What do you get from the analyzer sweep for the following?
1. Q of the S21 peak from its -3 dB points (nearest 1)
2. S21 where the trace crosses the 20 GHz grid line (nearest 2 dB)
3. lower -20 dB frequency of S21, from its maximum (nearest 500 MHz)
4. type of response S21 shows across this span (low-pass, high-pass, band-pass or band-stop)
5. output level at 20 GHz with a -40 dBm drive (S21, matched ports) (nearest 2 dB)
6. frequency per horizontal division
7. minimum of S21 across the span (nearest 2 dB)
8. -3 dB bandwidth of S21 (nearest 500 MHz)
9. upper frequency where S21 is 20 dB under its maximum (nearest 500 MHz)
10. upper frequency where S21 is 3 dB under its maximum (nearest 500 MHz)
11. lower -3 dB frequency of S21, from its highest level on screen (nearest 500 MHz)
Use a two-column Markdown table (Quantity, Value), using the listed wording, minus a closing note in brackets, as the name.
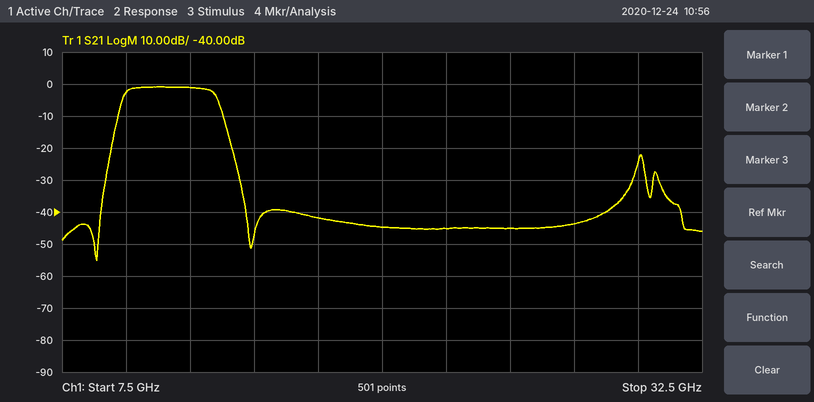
| Quantity | Value |
|---|---|
| Q of the S21 peak from its -3 dB points | 3 |
| S21 where the trace crosses the 20 GHz grid line | -44 dB |
| lower -20 dB frequency of S21, from its maximum | 9.5 GHz |
| type of response S21 shows across this span | band-pass |
| output level at 20 GHz with a -40 dBm drive (S21, matched ports) | -84 dBm |
| frequency per horizontal division | 2.5 GHz |
| minimum of S21 across the span | -56 dB |
| -3 dB bandwidth of S21 | 3.5 GHz |
| upper frequency where S21 is 20 dB under its maximum | 14.0 GHz |
| upper frequency where S21 is 3 dB under its maximum | 13.5 GHz |
| lower -3 dB frequency of S21, from its highest level on screen | 10.0 GHz |
